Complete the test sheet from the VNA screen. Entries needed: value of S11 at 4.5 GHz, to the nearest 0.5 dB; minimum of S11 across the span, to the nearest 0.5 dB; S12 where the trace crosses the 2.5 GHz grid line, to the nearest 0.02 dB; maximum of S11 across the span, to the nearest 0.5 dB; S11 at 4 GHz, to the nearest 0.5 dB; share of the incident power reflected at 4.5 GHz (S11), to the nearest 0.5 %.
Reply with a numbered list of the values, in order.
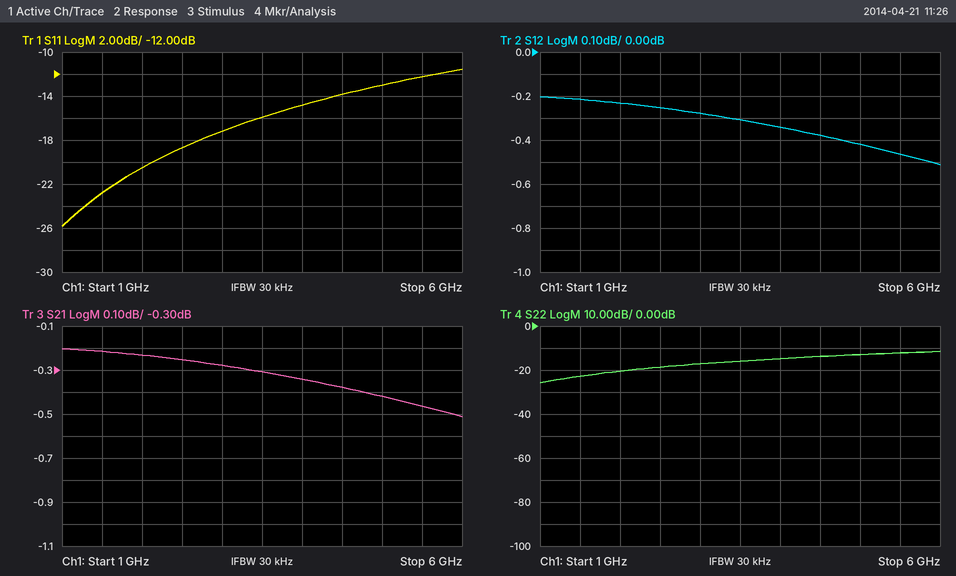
1. -14.0 dB
2. -26.0 dB
3. -0.26 dB
4. -11.5 dB
5. -15.0 dB
6. 4.0 %
